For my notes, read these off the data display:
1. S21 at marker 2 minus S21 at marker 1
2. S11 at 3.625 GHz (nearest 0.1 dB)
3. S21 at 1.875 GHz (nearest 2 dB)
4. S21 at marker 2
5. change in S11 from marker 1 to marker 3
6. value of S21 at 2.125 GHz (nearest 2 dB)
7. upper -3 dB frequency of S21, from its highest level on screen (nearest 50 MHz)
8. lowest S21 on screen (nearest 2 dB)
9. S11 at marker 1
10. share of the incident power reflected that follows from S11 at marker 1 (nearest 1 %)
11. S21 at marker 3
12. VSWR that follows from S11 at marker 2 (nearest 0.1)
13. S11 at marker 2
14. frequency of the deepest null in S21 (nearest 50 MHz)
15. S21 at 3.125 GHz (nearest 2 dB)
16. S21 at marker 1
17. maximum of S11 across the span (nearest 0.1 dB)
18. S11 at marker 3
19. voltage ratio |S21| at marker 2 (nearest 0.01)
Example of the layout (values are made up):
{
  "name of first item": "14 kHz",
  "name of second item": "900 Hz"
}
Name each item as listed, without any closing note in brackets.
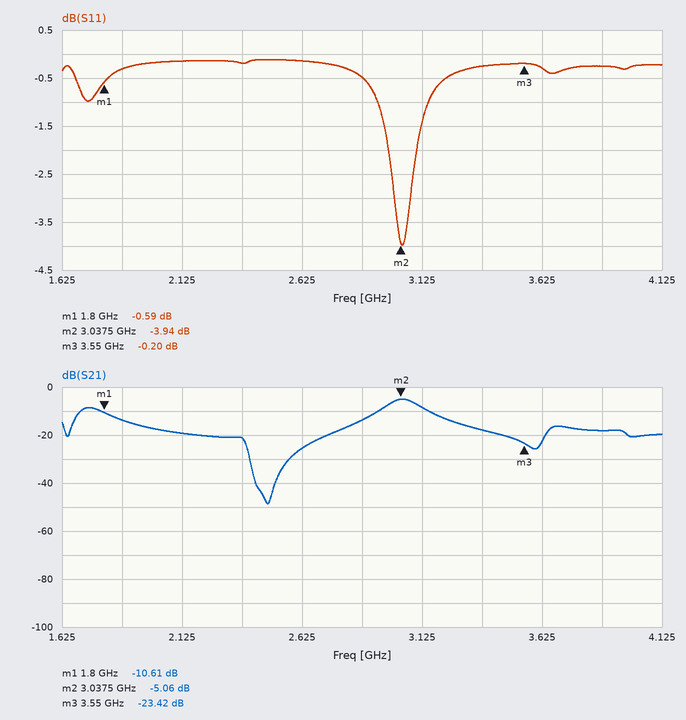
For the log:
{
  "S21 at marker 2 minus S21 at marker 1": "5.55 dB",
  "S11 at 3.625 GHz": "-0.3 dB",
  "S21 at 1.875 GHz": "-14 dB",
  "S21 at marker 2": "-5.06 dB",
  "change in S11 from marker 1 to marker 3": "0.39 dB",
  "value of S21 at 2.125 GHz": "-20 dB",
  "upper -3 dB frequency of S21, from its highest level on screen": "3.10 GHz",
  "lowest S21 on screen": "-48 dB",
  "S11 at marker 1": "-0.59 dB",
  "share of the incident power reflected that follows from S11 at marker 1": "87 %",
  "S21 at marker 3": "-23.42 dB",
  "VSWR that follows from S11 at marker 2": "4.5",
  "S11 at marker 2": "-3.94 dB",
  "frequency of the deepest null in S21": "2.50 GHz",
  "S21 at 3.125 GHz": "-8 dB",
  "S21 at marker 1": "-10.61 dB",
  "maximum of S11 across the span": "-0.1 dB",
  "S11 at marker 3": "-0.20 dB",
  "voltage ratio |S21| at marker 2": "0.56"
}
